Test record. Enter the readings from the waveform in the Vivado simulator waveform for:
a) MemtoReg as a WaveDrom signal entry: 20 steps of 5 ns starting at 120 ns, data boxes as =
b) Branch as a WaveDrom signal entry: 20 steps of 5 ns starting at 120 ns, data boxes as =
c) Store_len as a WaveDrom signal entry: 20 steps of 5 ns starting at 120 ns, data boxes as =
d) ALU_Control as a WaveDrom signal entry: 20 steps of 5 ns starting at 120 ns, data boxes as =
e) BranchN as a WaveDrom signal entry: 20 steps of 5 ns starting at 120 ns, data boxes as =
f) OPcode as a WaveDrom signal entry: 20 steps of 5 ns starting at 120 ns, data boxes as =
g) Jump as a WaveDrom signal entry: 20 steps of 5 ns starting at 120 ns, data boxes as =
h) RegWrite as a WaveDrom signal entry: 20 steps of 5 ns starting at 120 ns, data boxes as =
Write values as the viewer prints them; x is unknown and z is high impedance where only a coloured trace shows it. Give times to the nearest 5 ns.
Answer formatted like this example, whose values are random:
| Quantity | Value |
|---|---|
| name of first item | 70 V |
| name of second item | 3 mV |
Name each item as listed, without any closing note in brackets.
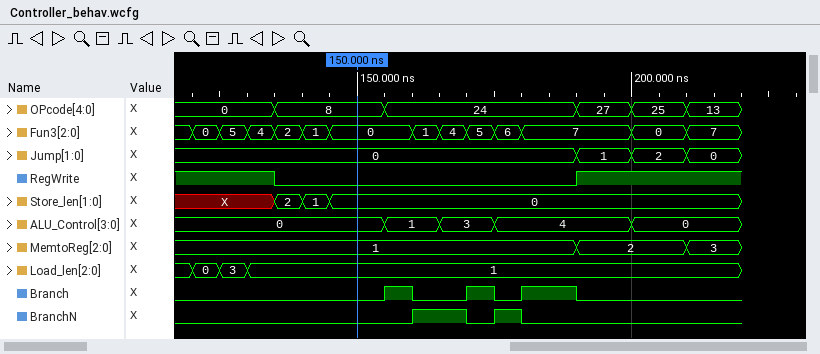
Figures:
| Quantity | Value |
|---|---|
| MemtoReg as a WaveDrom signal entry: 20 steps of 5 ns starting at 120 ns, data boxes as = | {name: 'MemtoReg', wave: '=.............=...=.', data: '1 2 3'} |
| Branch as a WaveDrom signal entry: 20 steps of 5 ns starting at 120 ns, data boxes as = | {name: 'Branch', wave: '0......10.101.0.....'} |
| Store_len as a WaveDrom signal entry: 20 steps of 5 ns starting at 120 ns, data boxes as = | {name: 'Store_len', wave: 'x..===..............', data: '2 1 0'} |
| ALU_Control as a WaveDrom signal entry: 20 steps of 5 ns starting at 120 ns, data boxes as = | {name: 'ALU_Control', wave: '=......=.=.=....=...', data: '0 1 3 4 0'} |
| BranchN as a WaveDrom signal entry: 20 steps of 5 ns starting at 120 ns, data boxes as = | {name: 'BranchN', wave: '0.......1.010.......'} |
| OPcode as a WaveDrom signal entry: 20 steps of 5 ns starting at 120 ns, data boxes as = | {name: 'OPcode', wave: '=..=...=......=.=.=.', data: '0 8 24 27 25 13'} |
| Jump as a WaveDrom signal entry: 20 steps of 5 ns starting at 120 ns, data boxes as = | {name: 'Jump', wave: '=.............=.=.=.', data: '0 1 2 0'} |
| RegWrite as a WaveDrom signal entry: 20 steps of 5 ns starting at 120 ns, data boxes as = | {name: 'RegWrite', wave: '1..0..........1.....'} |
